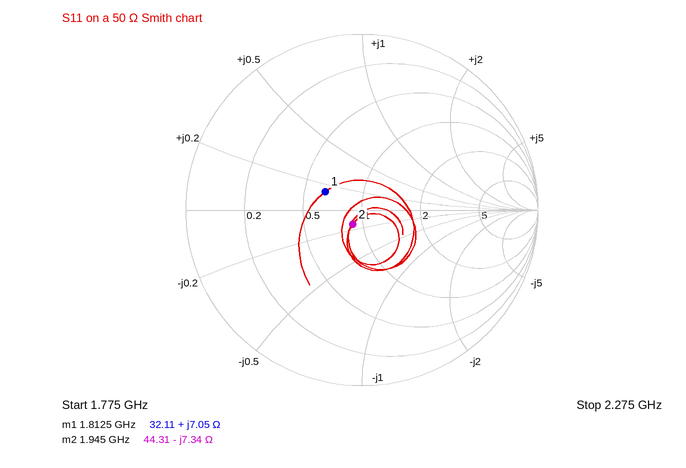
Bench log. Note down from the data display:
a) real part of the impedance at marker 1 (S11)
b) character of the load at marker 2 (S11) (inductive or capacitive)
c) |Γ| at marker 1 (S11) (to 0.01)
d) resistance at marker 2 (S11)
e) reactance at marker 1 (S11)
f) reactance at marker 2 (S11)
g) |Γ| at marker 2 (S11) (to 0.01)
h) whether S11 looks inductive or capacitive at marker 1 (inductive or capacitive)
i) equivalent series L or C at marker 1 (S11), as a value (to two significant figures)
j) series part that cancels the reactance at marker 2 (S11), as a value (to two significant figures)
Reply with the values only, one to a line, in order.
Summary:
32.11 Ω
capacitive
0.23
44.31 Ω
+7.05 Ω
-7.34 Ω
0.10
inductive
620 pH
600 pH
